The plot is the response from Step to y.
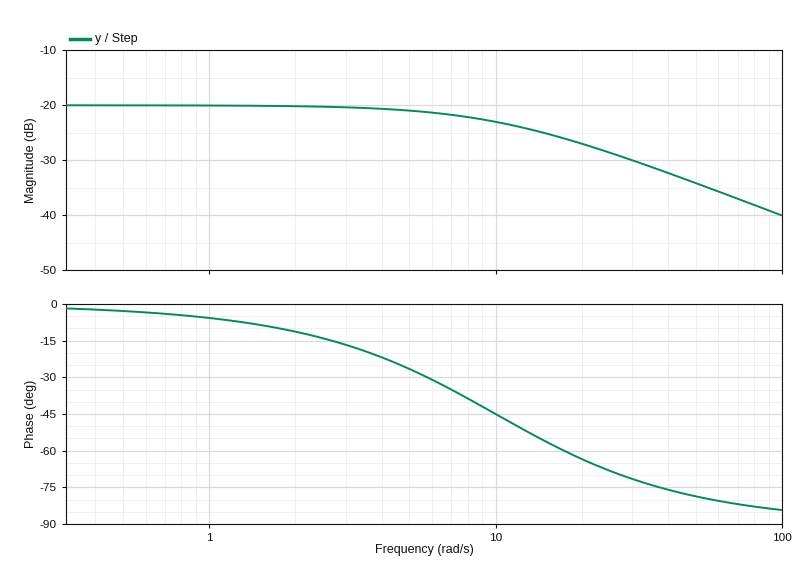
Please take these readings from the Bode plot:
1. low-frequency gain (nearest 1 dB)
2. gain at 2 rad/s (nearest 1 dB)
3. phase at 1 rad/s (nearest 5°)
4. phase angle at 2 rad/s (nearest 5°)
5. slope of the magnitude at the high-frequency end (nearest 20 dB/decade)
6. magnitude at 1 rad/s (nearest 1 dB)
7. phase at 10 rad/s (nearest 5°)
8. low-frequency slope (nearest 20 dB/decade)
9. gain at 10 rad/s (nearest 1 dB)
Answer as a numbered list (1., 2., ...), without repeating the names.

1. -20 dB
2. -20 dB
3. -5°
4. -10°
5. -20 dB/decade
6. -20 dB
7. -45°
8. 0 dB/decade
9. -23 dB
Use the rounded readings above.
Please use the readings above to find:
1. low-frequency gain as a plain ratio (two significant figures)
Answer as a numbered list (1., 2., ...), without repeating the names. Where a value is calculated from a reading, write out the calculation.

1. 10^(-20 / 20) = 0.10
